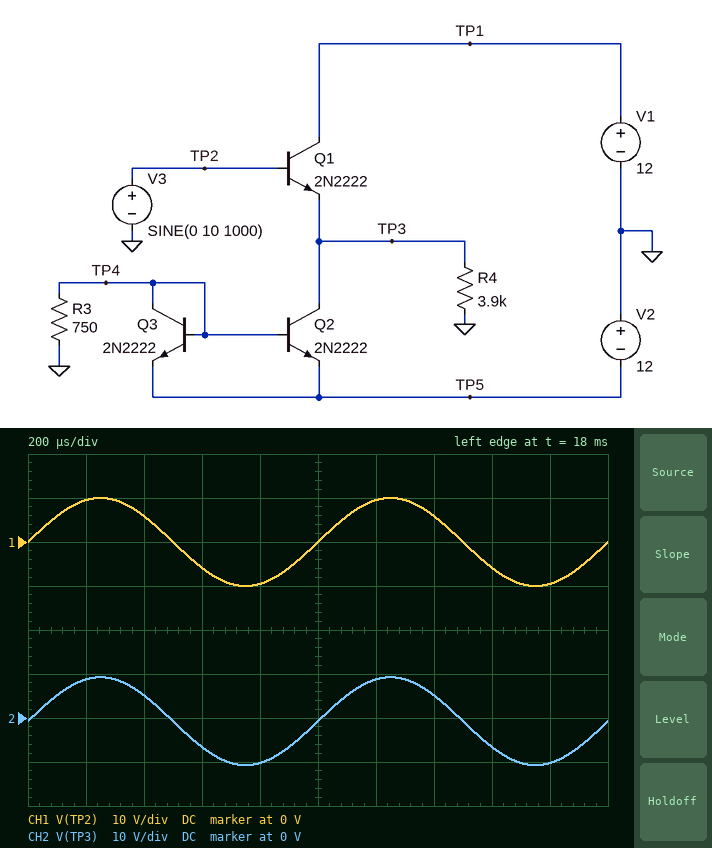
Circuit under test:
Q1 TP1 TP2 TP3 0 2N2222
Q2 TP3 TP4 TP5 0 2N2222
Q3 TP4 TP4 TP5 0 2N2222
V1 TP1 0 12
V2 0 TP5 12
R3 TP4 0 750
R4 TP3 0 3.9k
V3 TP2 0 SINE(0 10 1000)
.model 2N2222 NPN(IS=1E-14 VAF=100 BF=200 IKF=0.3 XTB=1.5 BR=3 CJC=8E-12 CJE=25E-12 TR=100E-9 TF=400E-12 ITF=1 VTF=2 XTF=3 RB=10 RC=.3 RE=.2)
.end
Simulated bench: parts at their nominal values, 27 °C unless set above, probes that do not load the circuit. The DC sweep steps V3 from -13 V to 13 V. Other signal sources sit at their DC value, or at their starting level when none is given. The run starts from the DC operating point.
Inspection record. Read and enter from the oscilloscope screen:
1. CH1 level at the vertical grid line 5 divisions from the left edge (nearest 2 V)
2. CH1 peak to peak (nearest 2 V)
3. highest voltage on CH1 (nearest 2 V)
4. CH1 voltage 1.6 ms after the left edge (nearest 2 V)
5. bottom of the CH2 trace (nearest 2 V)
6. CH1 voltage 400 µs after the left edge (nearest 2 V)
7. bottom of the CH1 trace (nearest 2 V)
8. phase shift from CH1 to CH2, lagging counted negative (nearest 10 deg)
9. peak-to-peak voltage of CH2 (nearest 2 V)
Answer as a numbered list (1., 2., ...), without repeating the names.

1. 0 V
2. 20 V
3. 10 V
4. -6 V
5. -10 V
6. 6 V
7. -10 V
8. 0 deg
9. 20 V
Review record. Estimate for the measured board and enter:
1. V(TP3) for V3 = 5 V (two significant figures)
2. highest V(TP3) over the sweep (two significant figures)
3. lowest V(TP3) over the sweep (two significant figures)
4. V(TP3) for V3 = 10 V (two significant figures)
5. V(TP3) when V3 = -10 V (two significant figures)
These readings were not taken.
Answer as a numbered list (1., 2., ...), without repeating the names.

1. 4.3 V
2. 12 V
3. -12 V
4. 9.3 V
5. -11 V
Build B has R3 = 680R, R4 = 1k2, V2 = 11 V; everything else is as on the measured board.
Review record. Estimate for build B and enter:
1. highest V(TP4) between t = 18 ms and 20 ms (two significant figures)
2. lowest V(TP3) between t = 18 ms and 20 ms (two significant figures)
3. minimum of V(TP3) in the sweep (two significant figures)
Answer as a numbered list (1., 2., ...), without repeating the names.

1. -10 V
2. -11 V
3. -11 V
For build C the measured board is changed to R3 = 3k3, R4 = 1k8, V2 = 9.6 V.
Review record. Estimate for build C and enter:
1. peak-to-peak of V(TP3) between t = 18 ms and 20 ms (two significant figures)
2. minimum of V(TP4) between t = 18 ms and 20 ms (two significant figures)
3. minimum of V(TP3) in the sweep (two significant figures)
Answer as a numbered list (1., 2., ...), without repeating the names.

1. 14 V
2. -8.9 V
3. -5.0 V
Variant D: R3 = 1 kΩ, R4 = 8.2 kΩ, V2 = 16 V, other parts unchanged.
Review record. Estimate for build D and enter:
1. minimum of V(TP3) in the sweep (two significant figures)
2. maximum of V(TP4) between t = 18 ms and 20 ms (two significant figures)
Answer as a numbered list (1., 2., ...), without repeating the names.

1. -14 V
2. -15 V
